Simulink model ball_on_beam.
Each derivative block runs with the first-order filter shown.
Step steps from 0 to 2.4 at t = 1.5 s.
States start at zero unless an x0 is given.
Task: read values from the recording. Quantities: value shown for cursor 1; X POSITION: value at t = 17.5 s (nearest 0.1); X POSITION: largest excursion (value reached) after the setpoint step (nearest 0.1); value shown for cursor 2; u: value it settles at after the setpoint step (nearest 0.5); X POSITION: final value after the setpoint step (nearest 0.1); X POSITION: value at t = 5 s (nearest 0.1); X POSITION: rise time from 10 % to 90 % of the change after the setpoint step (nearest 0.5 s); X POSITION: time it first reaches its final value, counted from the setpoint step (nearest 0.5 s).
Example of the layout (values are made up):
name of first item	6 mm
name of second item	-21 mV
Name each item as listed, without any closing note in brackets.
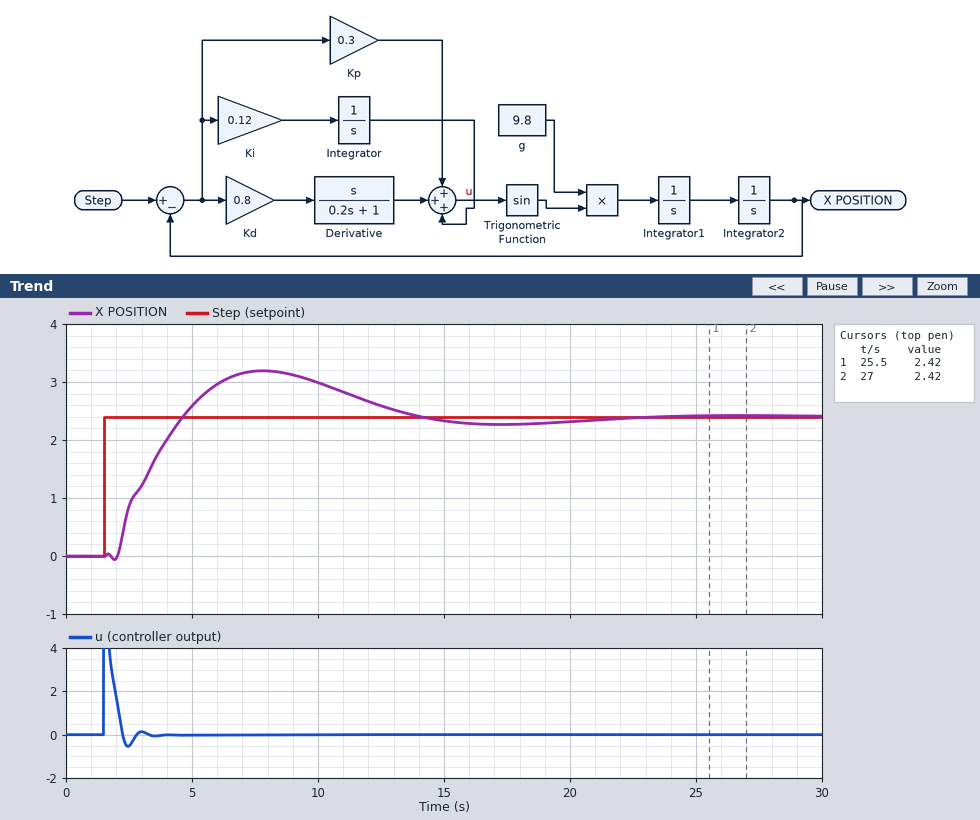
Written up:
value shown for cursor 1	2.42
X POSITION: value at t = 17.5 s	2.3
X POSITION: largest excursion (value reached) after the setpoint step	3.2
value shown for cursor 2	2.42
u: value it settles at after the setpoint step	0.0
X POSITION: final value after the setpoint step	2.4
X POSITION: value at t = 5 s	2.6
X POSITION: rise time from 10 % to 90 % of the change after the setpoint step	2.0 s
X POSITION: time it first reaches its final value, counted from the setpoint step	3.0 s
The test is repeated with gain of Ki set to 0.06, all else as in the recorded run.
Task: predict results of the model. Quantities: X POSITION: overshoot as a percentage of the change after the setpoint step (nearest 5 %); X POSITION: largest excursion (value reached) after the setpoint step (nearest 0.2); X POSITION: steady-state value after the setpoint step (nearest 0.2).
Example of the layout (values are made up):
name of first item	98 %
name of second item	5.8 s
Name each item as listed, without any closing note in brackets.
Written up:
X POSITION: overshoot as a percentage of the change after the setpoint step	25 %
X POSITION: largest excursion (value reached) after the setpoint step	3.0
X POSITION: steady-state value after the setpoint step	2.4
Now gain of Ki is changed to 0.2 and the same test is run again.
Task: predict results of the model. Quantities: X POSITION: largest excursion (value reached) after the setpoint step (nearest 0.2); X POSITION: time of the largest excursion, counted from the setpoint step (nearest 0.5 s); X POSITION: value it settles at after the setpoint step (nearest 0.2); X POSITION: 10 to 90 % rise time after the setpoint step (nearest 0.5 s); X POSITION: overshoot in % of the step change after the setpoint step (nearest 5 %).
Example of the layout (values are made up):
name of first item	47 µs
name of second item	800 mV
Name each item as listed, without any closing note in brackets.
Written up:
X POSITION: largest excursion (value reached) after the setpoint step	3.4
X POSITION: time of the largest excursion, counted from the setpoint step	5.0 s
X POSITION: value it settles at after the setpoint step	2.4
X POSITION: 10 to 90 % rise time after the setpoint step	1.5 s
X POSITION: overshoot in % of the step change after the setpoint step	40 %
